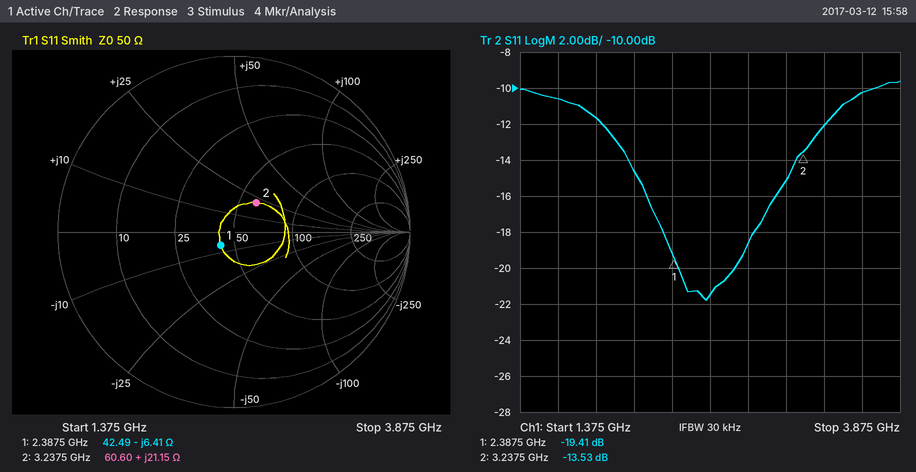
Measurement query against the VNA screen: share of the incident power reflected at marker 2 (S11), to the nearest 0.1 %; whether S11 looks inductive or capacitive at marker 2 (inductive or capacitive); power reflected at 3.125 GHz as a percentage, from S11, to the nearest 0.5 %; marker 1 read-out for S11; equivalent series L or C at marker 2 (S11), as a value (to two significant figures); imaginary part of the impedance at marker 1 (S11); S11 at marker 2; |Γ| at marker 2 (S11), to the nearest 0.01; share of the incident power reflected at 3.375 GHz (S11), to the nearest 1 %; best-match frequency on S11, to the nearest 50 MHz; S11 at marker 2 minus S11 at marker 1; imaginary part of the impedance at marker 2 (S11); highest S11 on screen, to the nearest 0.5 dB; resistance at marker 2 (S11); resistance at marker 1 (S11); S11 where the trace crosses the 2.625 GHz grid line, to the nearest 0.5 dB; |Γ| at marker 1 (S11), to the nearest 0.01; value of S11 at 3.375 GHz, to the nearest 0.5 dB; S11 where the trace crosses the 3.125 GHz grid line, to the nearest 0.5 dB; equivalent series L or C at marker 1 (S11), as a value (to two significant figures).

4.4 %
inductive
3.0 %
-19.41 dB
1.0 nH
-6.41 Ω
-13.53 dB
0.21
6 %
2.60 GHz
5.88 dB
+21.15 Ω
-9.5 dB
60.60 Ω
42.49 Ω
-21.5 dB
0.11
-12.0 dB
-15.0 dB
10 pF
